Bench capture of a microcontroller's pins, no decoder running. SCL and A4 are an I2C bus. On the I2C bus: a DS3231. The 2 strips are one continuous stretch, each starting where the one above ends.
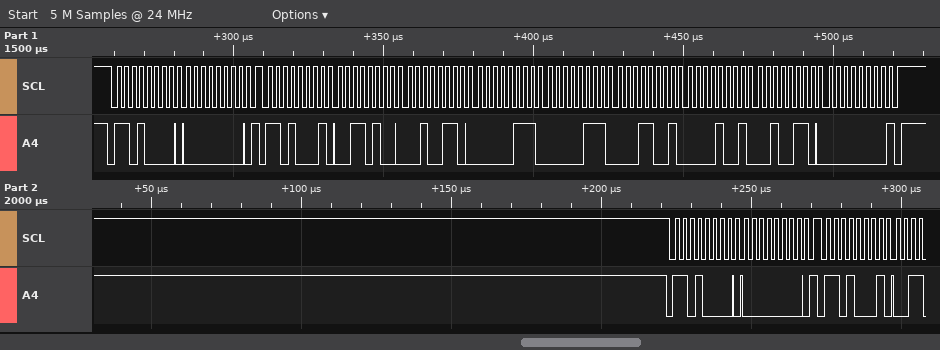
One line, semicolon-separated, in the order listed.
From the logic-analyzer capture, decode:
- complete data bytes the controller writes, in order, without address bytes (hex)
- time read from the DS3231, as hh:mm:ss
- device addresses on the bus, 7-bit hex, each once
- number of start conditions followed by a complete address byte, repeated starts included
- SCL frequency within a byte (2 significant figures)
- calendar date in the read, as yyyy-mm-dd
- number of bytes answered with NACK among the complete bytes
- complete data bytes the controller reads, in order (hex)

00 00; 07:26:34; 0x68; 4; 400 kHz; 2026-09-19; 1; 34 26 07 07 19 09 26 00
